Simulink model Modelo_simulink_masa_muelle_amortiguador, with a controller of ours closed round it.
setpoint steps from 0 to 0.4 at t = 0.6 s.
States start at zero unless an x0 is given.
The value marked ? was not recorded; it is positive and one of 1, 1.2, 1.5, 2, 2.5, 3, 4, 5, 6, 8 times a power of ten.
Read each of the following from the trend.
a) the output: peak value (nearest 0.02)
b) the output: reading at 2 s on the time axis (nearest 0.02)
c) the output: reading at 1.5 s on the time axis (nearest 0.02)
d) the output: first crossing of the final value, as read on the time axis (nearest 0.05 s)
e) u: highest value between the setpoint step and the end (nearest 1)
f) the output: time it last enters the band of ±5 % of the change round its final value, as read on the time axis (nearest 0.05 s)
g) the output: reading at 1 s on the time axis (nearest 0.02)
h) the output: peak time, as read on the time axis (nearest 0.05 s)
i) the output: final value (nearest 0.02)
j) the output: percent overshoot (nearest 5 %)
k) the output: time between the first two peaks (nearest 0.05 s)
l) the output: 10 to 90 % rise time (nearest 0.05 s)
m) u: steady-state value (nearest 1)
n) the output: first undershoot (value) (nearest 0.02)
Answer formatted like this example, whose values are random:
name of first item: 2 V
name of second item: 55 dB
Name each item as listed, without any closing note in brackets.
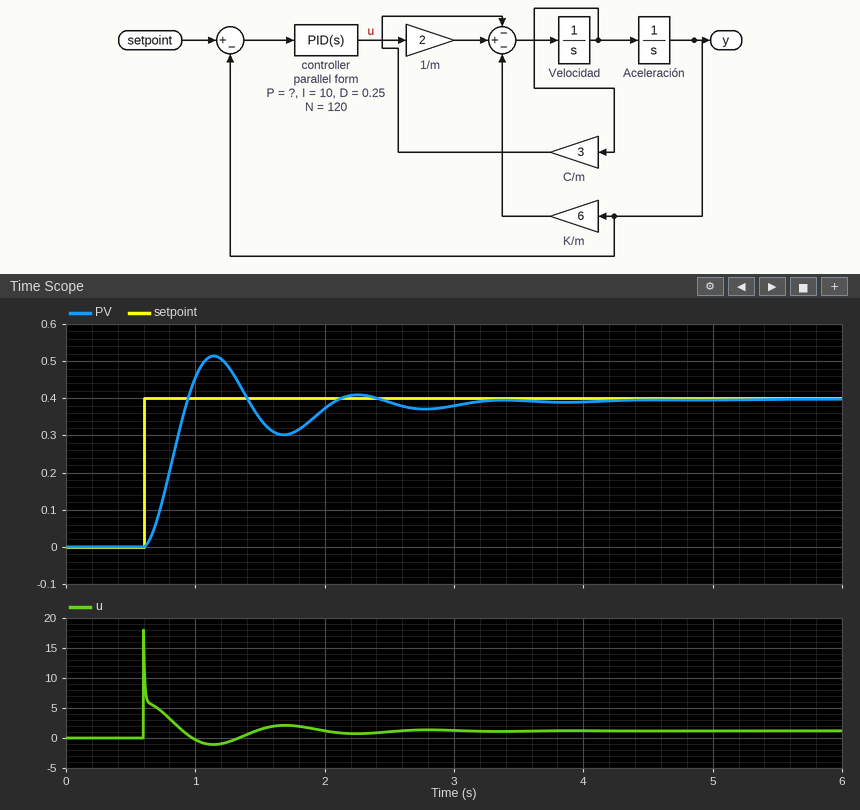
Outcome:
the output: peak value: 0.52
the output: reading at 2 s on the time axis: 0.38
the output: reading at 1.5 s on the time axis: 0.34
the output: first crossing of the final value, as read on the time axis: 0.95 s
u: highest value between the setpoint step and the end: 18
the output: time it last enters the band of ±5 % of the change round its final value, as read on the time axis: 3.00 s
the output: reading at 1 s on the time axis: 0.46
the output: peak time, as read on the time axis: 1.15 s
the output: final value: 0.40
the output: percent overshoot: 30 %
the output: time between the first two peaks: 1.10 s
the output: 10 to 90 % rise time: 0.25 s
u: steady-state value: 1
the output: first undershoot (value): 0.30
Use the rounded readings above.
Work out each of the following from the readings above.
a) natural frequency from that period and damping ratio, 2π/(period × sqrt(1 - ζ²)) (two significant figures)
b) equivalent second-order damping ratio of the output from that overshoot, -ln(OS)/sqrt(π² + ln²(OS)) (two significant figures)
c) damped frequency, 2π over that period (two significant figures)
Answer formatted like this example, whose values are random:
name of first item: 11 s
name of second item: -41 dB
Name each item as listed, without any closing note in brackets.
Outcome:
natural frequency from that period and damping ratio, 2π/(period × sqrt(1 - ζ²)): 6.1 rad/s
equivalent second-order damping ratio of the output from that overshoot, -ln(OS)/sqrt(π² + ln²(OS)): 0.36
damped frequency, 2π over that period: 5.7 rad/s
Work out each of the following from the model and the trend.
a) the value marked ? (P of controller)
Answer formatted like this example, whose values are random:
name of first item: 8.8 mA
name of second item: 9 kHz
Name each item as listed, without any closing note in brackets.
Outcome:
the value marked ?: 15
